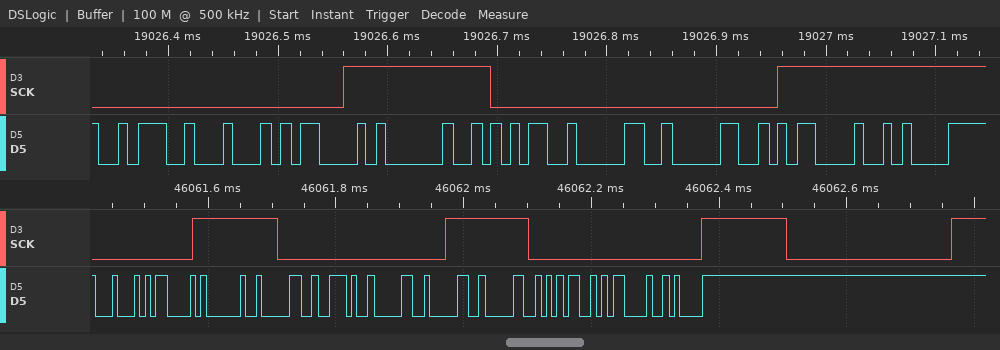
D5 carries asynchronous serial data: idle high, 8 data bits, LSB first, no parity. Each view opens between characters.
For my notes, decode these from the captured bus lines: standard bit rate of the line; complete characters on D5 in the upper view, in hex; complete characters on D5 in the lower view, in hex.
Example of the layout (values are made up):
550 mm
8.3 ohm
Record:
115200 baud
3A, 44, 43, 20, 35, 30, 30, 0D, 0A
44, 43, 20, 30, 2E, 30, 30, 30, 35, 0D, 0A
